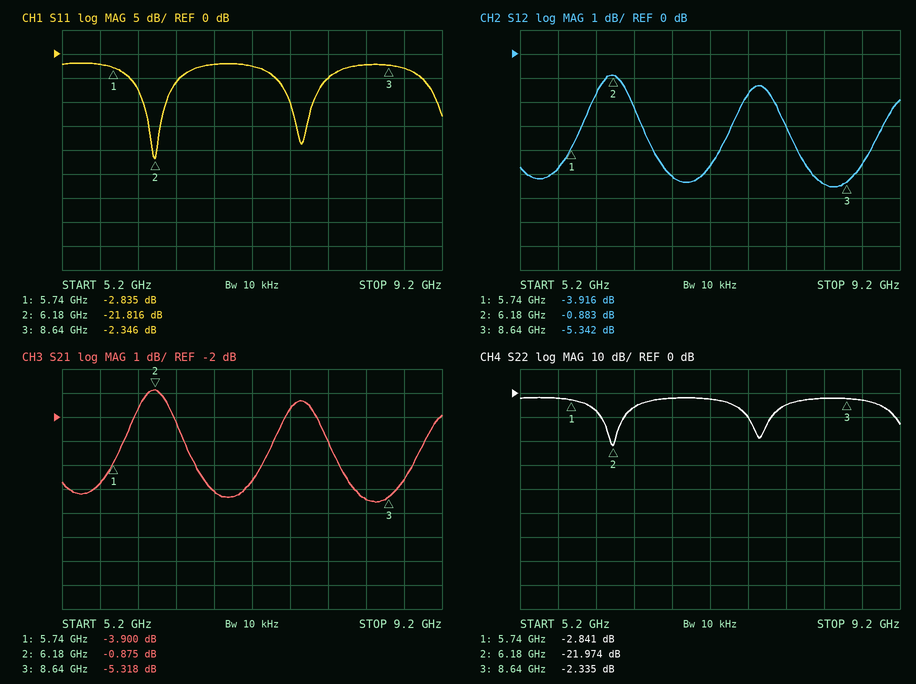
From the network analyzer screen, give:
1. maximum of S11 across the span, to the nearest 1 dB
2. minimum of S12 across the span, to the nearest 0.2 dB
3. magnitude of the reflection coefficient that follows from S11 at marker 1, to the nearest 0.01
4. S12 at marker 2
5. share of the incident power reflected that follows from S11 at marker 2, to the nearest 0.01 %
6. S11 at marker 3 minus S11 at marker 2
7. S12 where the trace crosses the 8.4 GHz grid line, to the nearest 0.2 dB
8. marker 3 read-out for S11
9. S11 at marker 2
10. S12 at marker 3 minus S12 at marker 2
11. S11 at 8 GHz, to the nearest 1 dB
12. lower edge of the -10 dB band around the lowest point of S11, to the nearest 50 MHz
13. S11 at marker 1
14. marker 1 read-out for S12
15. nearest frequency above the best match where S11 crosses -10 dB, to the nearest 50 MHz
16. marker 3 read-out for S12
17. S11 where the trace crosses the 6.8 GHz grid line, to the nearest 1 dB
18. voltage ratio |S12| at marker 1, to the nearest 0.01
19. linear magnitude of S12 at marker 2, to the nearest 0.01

-2 dB
-5.6 dB
0.72
-0.883 dB
0.66 %
19.470 dB
-5.4 dB
-2.346 dB
-21.816 dB
-4.459 dB
-5 dB
6.05 GHz
-2.835 dB
-3.916 dB
6.30 GHz
-5.342 dB
-2 dB
0.64
0.90
